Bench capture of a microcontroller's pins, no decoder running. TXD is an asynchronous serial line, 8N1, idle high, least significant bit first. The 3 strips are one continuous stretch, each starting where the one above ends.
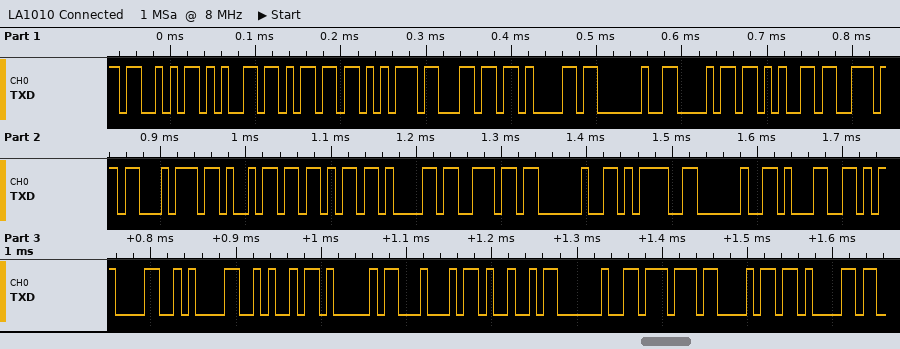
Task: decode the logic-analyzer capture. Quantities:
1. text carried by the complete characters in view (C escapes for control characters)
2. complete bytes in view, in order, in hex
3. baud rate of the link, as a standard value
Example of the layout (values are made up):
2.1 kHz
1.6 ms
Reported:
"Semula hentikan = 1\r\nJADI wha"
0x53 0x65 0x6D 0x75 0x6C 0x61 0x20 0x68 0x65 0x6E 0x74 0x69 0x6B 0x61 0x6E 0x20 0x3D 0x20 0x31 0x0D 0x0A 0x4A 0x41 0x44 0x49 0x20 0x77 0x68 0x61
115200 baud
